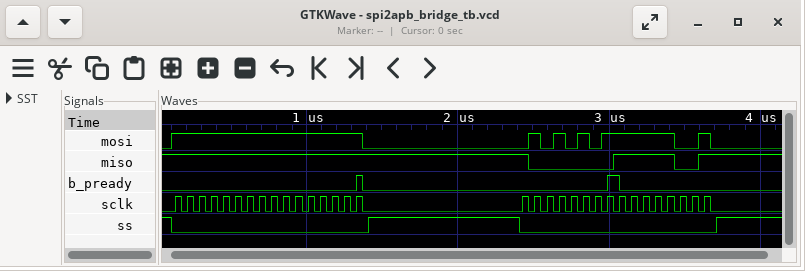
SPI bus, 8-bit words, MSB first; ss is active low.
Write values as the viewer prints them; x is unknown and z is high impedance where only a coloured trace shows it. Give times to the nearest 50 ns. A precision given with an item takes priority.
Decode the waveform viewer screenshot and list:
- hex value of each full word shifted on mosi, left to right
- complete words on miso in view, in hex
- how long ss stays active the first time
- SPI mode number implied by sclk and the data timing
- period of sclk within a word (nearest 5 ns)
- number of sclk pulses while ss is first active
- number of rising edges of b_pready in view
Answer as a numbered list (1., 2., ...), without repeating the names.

1. FF, FF, 55, F9
2. FF, FF, 80, F9
3. 1300 ns
4. 0
5. 80 ns
6. 16
7. 2
